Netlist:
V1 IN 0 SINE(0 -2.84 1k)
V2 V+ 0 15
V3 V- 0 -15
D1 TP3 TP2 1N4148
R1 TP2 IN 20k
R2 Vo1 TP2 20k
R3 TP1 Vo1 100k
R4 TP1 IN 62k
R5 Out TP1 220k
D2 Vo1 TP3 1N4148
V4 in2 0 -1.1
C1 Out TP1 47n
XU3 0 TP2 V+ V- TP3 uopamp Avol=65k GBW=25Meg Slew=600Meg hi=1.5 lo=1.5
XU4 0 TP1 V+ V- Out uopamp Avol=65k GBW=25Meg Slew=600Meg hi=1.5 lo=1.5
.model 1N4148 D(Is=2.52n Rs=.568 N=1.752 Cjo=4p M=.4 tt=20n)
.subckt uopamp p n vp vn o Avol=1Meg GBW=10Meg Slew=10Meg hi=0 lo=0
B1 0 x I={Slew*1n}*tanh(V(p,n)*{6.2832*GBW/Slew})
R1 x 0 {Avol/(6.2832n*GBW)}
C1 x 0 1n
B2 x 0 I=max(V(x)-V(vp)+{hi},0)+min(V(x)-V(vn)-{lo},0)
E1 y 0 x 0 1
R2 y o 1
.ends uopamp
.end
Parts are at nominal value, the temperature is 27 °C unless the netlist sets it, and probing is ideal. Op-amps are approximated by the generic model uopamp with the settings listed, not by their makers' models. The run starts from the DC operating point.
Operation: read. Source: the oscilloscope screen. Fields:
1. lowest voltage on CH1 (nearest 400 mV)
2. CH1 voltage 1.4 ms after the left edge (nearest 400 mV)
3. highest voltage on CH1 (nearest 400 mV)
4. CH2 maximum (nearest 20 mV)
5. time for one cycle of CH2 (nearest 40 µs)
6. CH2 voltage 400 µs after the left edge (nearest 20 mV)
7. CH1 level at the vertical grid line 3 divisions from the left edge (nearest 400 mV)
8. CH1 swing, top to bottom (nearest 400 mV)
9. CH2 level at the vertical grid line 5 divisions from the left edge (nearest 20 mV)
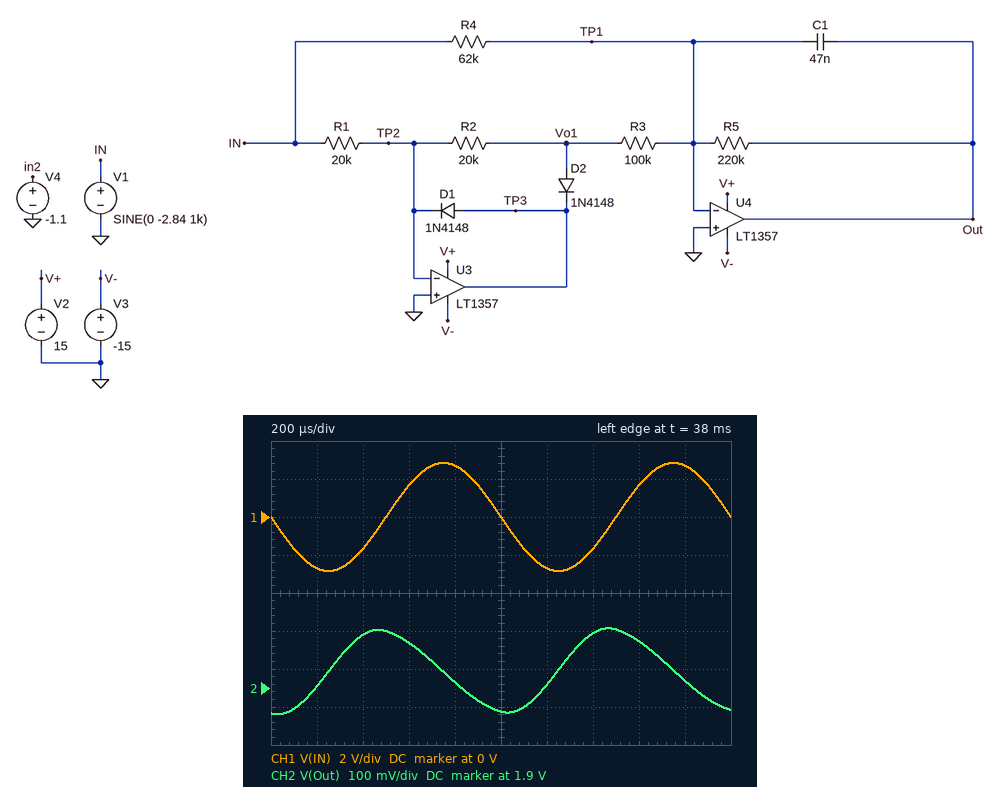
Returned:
-2.8 V
-1.6 V
2.8 V
2.06 V
1.00 ms
2.04 V
1.6 V
5.6 V
1.84 V
